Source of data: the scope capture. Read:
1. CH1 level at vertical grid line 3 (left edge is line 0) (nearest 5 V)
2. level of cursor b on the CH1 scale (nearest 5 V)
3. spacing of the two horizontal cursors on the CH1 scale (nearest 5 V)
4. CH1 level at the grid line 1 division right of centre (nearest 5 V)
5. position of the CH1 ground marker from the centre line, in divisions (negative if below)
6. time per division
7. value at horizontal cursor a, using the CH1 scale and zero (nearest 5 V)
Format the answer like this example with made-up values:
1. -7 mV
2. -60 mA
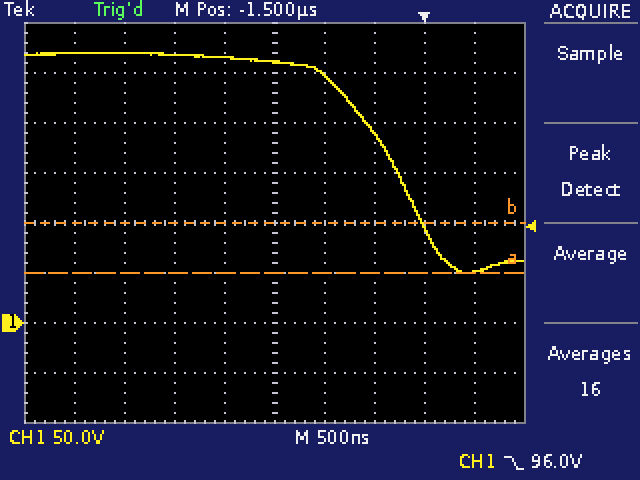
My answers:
1. 270 V
2. 100 V
3. 50 V
4. 250 V
5. -2.0 div
6. 500 ns
7. 50 V
